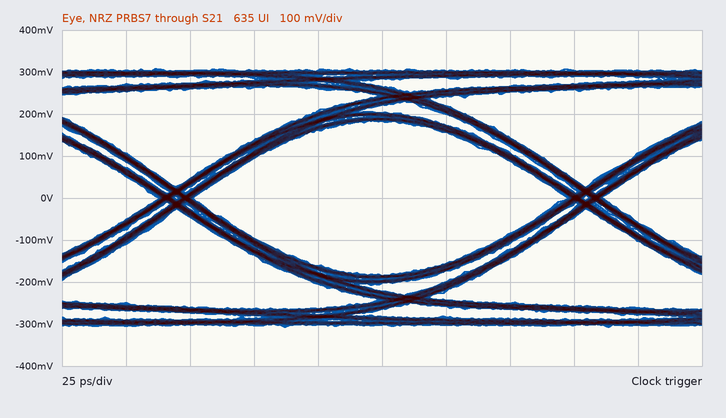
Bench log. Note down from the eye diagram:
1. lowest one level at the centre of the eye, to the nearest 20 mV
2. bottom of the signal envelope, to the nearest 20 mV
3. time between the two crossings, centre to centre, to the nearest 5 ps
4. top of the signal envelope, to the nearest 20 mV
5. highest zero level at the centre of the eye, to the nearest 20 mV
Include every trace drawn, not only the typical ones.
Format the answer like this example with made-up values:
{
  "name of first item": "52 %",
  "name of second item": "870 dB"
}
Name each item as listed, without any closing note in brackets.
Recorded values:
{
  "lowest one level at the centre of the eye, to the nearest 20 mV": "180 mV",
  "bottom of the signal envelope, to the nearest 20 mV": "-300 mV",
  "time between the two crossings, centre to centre, to the nearest 5 ps": "160 ps",
  "top of the signal envelope, to the nearest 20 mV": "300 mV",
  "highest zero level at the centre of the eye, to the nearest 20 mV": "-180 mV"
}
